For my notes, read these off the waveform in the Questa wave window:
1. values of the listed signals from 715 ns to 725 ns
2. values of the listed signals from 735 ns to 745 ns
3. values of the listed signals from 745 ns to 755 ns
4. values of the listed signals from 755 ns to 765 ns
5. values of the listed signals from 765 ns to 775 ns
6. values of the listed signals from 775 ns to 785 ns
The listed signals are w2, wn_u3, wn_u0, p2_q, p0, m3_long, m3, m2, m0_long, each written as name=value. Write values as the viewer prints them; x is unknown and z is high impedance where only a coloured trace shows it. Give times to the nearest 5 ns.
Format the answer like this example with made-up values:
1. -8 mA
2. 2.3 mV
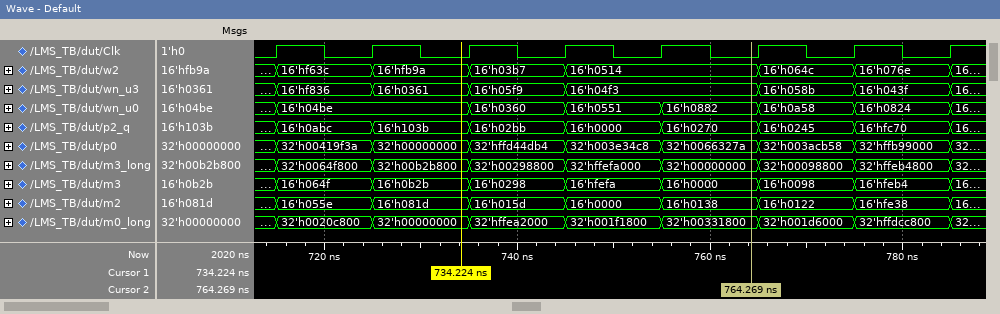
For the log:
1. w2=16'hf63c, wn_u3=16'hf836, wn_u0=16'h04be, p2_q=16'h0abc, p0=32'h00419f3a, m3_long=32'h0064f800, m3=16'h064f, m2=16'h055e, m0_long=32'h0020c800
2. w2=16'h03b7, wn_u3=16'h05f9, wn_u0=16'h0360, p2_q=16'h02bb, p0=32'hffd44db4, m3_long=32'h00298800, m3=16'h0298, m2=16'h015d, m0_long=32'hffea2000
3. w2=16'h0514, wn_u3=16'h04f3, wn_u0=16'h0551, p2_q=16'h0000, p0=32'h003e34c8, m3_long=32'hffefa000, m3=16'hfefa, m2=16'h0000, m0_long=32'h001f1800
4. w2=16'h0514, wn_u3=16'h04f3, wn_u0=16'h0882, p2_q=16'h0270, p0=32'h0066327a, m3_long=32'h00000000, m3=16'h0000, m2=16'h0138, m0_long=32'h00331800
5. w2=16'h064c, wn_u3=16'h058b, wn_u0=16'h0a58, p2_q=16'h0245, p0=32'h003acb58, m3_long=32'h00098800, m3=16'h0098, m2=16'h0122, m0_long=32'h001d6000
6. w2=16'h076e, wn_u3=16'h043f, wn_u0=16'h0824, p2_q=16'hfc70, p0=32'hffb99000, m3_long=32'hffeb4800, m3=16'hfeb4, m2=16'hfe38, m0_long=32'hffdcc800
